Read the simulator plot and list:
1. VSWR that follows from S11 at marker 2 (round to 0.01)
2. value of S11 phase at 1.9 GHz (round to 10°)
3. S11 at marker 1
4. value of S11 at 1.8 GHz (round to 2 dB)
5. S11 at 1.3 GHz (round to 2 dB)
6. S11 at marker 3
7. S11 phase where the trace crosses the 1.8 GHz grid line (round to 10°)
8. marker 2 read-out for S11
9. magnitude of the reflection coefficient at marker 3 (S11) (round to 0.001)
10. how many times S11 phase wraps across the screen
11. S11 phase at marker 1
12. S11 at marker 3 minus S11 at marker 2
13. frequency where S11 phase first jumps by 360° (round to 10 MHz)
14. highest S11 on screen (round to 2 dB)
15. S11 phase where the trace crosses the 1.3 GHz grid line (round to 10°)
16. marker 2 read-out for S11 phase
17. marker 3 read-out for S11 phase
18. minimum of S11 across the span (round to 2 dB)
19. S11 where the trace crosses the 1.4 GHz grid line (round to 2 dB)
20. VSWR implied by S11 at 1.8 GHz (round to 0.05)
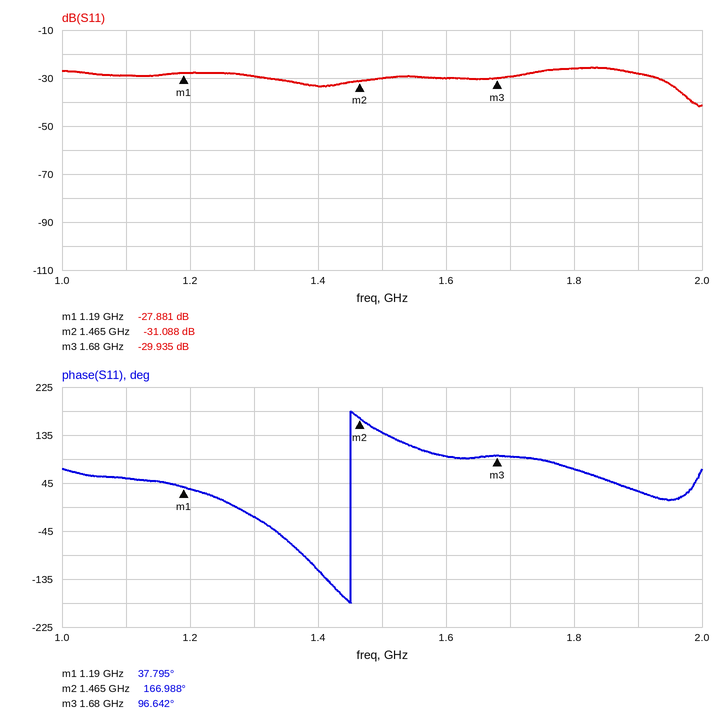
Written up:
1.06
30°
-27.881 dB
-26 dB
-30 dB
-29.935 dB
70°
-31.088 dB
0.032
1
37.795°
1.153 dB
1.45 GHz
-26 dB
-20°
166.988°
96.642°
-42 dB
-34 dB
1.10
